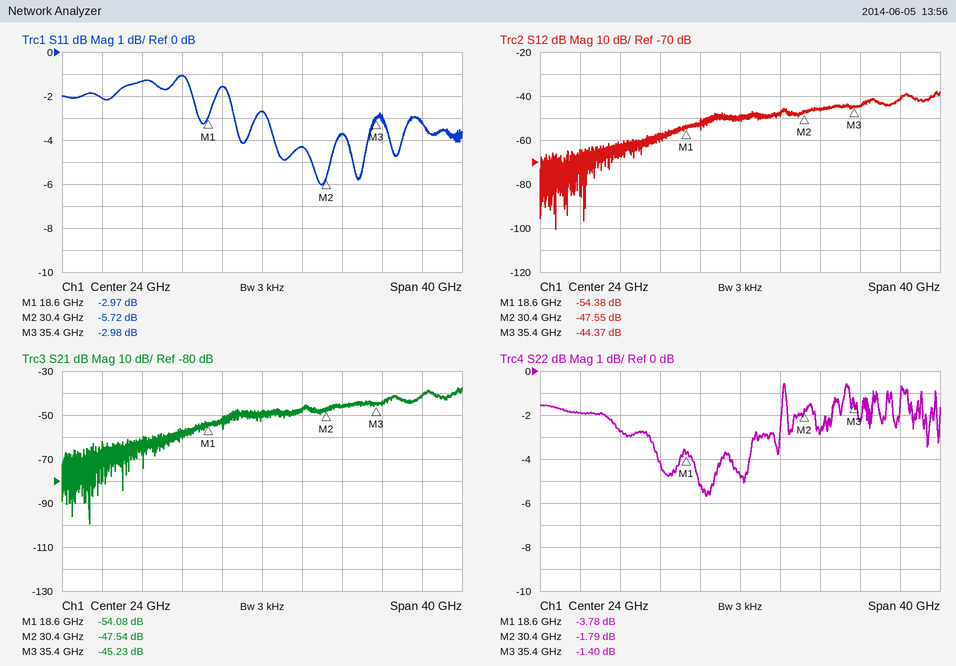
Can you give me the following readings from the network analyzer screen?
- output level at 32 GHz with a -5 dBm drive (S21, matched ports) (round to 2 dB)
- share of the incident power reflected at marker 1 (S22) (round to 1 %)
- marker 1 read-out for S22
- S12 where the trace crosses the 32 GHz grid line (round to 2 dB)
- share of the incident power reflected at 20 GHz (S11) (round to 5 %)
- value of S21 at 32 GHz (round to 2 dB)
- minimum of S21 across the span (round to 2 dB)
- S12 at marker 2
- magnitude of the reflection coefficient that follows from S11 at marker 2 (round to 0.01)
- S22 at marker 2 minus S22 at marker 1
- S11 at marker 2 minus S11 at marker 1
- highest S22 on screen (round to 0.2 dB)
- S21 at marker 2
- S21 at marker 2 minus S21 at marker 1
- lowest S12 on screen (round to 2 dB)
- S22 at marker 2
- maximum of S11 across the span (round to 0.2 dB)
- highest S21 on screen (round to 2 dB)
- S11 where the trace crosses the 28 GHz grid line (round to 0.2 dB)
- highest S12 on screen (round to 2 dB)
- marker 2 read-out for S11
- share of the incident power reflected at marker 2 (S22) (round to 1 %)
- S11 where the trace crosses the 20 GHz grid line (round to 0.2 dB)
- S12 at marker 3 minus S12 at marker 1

-50 dBm
42 %
-3.78 dB
-46 dB
70 %
-46 dB
-100 dB
-47.55 dB
0.52
1.99 dB
-2.75 dB
-0.6 dB
-47.54 dB
6.54 dB
-100 dB
-1.79 dB
-1.0 dB
-38 dB
-4.4 dB
-38 dB
-5.72 dB
66 %
-1.6 dB
10.01 dB
